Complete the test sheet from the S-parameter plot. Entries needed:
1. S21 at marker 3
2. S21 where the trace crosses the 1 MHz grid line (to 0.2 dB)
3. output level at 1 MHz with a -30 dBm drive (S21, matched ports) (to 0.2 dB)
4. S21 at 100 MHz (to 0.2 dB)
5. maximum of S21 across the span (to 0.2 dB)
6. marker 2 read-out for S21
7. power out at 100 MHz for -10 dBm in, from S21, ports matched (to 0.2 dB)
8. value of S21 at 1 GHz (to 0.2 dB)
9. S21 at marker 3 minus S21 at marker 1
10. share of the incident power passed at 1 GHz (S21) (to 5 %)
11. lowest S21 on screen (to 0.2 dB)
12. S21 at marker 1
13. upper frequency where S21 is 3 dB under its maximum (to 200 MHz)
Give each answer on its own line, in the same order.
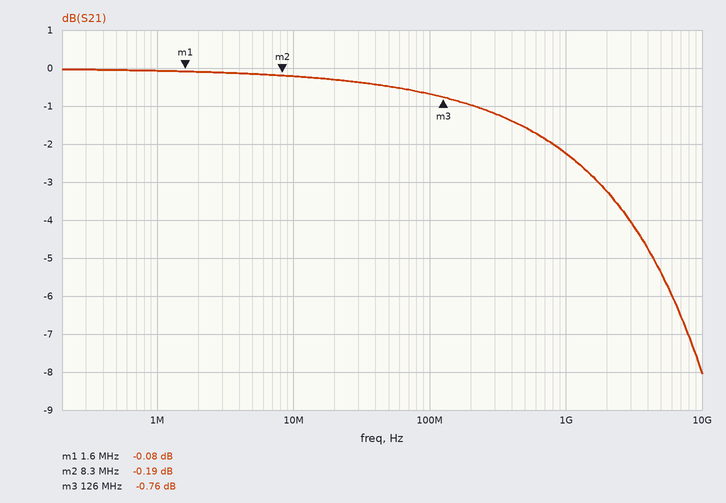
-0.76 dB
0.0 dB
-30.0 dBm
-0.6 dB
0.0 dB
-0.19 dB
-10.6 dBm
-2.2 dB
-0.68 dB
60 %
-8.0 dB
-0.08 dB
1.8 GHz
